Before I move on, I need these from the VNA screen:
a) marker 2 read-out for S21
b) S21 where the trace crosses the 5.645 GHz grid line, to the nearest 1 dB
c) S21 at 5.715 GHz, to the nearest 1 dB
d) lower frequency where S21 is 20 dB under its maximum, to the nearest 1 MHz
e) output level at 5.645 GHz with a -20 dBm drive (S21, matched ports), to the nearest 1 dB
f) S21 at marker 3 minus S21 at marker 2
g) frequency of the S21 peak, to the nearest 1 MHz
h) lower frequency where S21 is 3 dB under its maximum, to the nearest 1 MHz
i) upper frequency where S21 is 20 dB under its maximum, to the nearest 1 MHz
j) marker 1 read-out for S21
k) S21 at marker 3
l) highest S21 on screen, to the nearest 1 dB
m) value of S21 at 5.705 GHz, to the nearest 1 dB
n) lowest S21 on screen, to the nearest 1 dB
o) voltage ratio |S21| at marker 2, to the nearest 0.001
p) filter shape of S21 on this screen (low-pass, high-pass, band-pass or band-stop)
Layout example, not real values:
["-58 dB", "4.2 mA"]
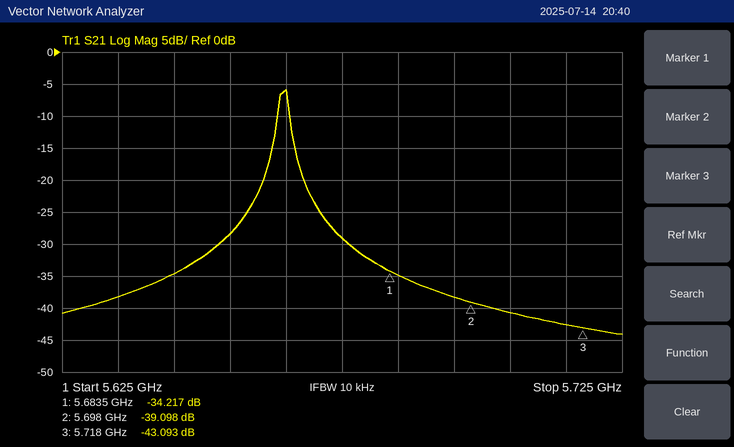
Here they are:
["-39.098 dB", "-35 dB", "-43 dB", "5.657 GHz", "-55 dBm", "-3.995 dB", "5.665 GHz", "5.664 GHz", "5.672 GHz", "-34.217 dB", "-43.093 dB", "-6 dB", "-41 dB", "-44 dB", "0.011", "band-pass"]
